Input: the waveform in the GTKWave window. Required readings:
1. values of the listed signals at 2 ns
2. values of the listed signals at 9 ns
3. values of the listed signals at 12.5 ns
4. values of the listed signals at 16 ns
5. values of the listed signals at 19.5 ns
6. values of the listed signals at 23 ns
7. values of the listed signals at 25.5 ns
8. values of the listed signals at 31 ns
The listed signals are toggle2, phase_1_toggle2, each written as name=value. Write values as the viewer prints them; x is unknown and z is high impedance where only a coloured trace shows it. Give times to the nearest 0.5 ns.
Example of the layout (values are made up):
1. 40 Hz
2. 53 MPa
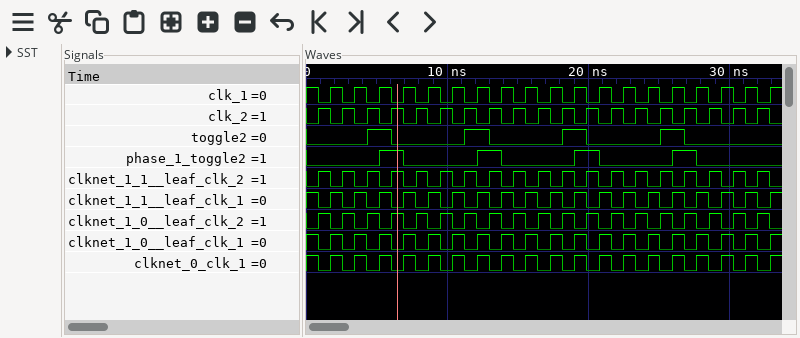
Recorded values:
1. toggle2=0, phase_1_toggle2=0
2. toggle2=0, phase_1_toggle2=0
3. toggle2=1, phase_1_toggle2=1
4. toggle2=0, phase_1_toggle2=0
5. toggle2=1, phase_1_toggle2=1
6. toggle2=0, phase_1_toggle2=0
7. toggle2=1, phase_1_toggle2=0
8. toggle2=0, phase_1_toggle2=0
